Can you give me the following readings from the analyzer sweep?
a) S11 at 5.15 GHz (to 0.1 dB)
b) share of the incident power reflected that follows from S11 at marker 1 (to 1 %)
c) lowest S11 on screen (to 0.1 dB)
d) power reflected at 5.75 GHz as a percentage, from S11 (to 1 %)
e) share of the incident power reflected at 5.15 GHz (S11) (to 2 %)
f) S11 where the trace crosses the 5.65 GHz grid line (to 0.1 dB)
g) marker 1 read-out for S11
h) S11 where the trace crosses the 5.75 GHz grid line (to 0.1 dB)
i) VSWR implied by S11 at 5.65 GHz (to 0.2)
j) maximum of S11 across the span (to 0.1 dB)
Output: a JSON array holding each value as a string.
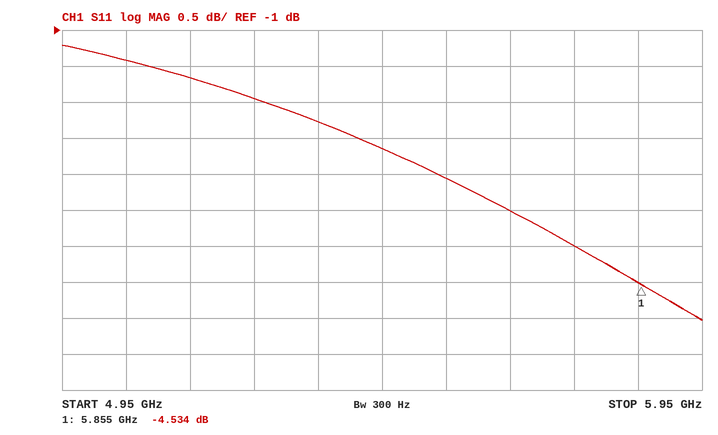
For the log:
["-1.7 dB", "35 %", "-5.0 dB", "40 %", "68 %", "-3.5 dB", "-4.534 dB", "-4.0 dB", "5.0", "-1.2 dB"]
